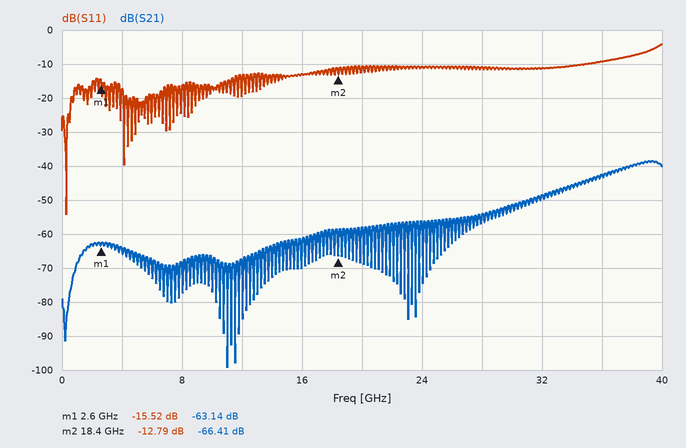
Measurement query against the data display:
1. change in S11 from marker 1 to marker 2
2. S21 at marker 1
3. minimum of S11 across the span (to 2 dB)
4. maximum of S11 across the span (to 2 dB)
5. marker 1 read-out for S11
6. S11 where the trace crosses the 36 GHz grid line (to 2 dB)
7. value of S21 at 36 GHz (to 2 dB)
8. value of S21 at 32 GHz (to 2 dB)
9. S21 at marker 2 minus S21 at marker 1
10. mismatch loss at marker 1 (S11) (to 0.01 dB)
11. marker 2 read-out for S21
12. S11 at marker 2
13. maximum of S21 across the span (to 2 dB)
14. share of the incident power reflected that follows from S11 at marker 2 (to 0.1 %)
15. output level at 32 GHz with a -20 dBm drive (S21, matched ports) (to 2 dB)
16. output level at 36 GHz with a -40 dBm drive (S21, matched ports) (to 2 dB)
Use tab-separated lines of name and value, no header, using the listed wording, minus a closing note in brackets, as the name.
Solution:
change in S11 from marker 1 to marker 2	2.73 dB
S21 at marker 1	-63.14 dB
minimum of S11 across the span	-54 dB
maximum of S11 across the span	-4 dB
marker 1 read-out for S11	-15.52 dB
S11 where the trace crosses the 36 GHz grid line	-10 dB
value of S21 at 36 GHz	-42 dB
value of S21 at 32 GHz	-48 dB
S21 at marker 2 minus S21 at marker 1	-3.27 dB
mismatch loss at marker 1 (S11)	0.12 dB
marker 2 read-out for S21	-66.41 dB
S11 at marker 2	-12.79 dB
maximum of S21 across the span	-38 dB
share of the incident power reflected that follows from S11 at marker 2	5.3 %
output level at 32 GHz with a -20 dBm drive (S21, matched ports)	-68 dBm
output level at 36 GHz with a -40 dBm drive (S21, matched ports)	-82 dBm
